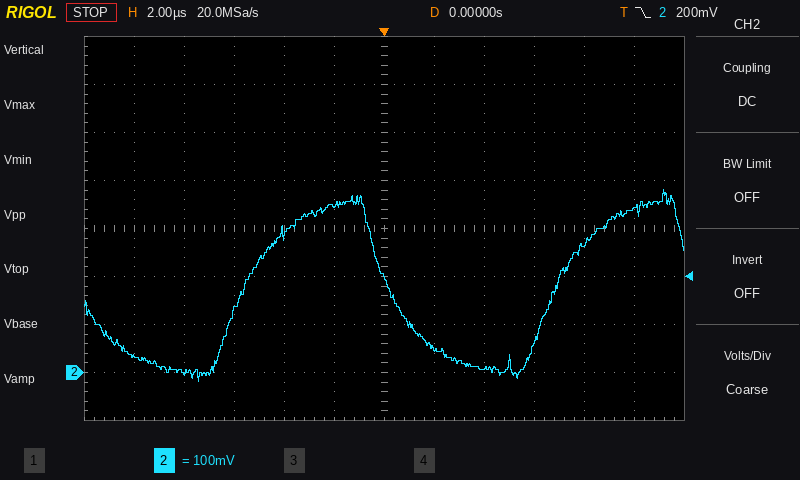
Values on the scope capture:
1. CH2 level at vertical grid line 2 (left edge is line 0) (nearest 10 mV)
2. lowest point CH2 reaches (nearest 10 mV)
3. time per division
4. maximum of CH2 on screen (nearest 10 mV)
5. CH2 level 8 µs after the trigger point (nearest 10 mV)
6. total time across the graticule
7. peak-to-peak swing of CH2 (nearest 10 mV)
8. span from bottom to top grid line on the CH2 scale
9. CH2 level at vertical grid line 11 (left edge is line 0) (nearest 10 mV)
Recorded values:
0 mV
-20 mV
2 µs
380 mV
270 mV
24 µs
400 mV
800 mV
340 mV
